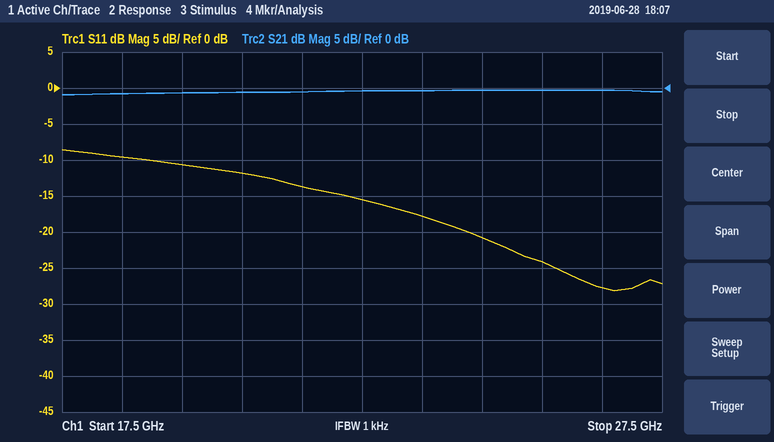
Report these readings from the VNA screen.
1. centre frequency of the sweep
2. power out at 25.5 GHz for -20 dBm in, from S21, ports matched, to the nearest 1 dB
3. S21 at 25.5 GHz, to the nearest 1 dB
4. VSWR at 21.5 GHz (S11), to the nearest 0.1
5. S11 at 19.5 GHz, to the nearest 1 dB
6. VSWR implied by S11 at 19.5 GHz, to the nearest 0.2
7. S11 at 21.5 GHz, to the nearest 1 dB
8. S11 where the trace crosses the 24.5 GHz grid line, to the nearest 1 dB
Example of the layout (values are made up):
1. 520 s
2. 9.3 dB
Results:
1. 22.5 GHz
2. -20 dBm
3. 0 dB
4. 1.5
5. -11 dB
6. 1.8
7. -14 dB
8. -21 dB
